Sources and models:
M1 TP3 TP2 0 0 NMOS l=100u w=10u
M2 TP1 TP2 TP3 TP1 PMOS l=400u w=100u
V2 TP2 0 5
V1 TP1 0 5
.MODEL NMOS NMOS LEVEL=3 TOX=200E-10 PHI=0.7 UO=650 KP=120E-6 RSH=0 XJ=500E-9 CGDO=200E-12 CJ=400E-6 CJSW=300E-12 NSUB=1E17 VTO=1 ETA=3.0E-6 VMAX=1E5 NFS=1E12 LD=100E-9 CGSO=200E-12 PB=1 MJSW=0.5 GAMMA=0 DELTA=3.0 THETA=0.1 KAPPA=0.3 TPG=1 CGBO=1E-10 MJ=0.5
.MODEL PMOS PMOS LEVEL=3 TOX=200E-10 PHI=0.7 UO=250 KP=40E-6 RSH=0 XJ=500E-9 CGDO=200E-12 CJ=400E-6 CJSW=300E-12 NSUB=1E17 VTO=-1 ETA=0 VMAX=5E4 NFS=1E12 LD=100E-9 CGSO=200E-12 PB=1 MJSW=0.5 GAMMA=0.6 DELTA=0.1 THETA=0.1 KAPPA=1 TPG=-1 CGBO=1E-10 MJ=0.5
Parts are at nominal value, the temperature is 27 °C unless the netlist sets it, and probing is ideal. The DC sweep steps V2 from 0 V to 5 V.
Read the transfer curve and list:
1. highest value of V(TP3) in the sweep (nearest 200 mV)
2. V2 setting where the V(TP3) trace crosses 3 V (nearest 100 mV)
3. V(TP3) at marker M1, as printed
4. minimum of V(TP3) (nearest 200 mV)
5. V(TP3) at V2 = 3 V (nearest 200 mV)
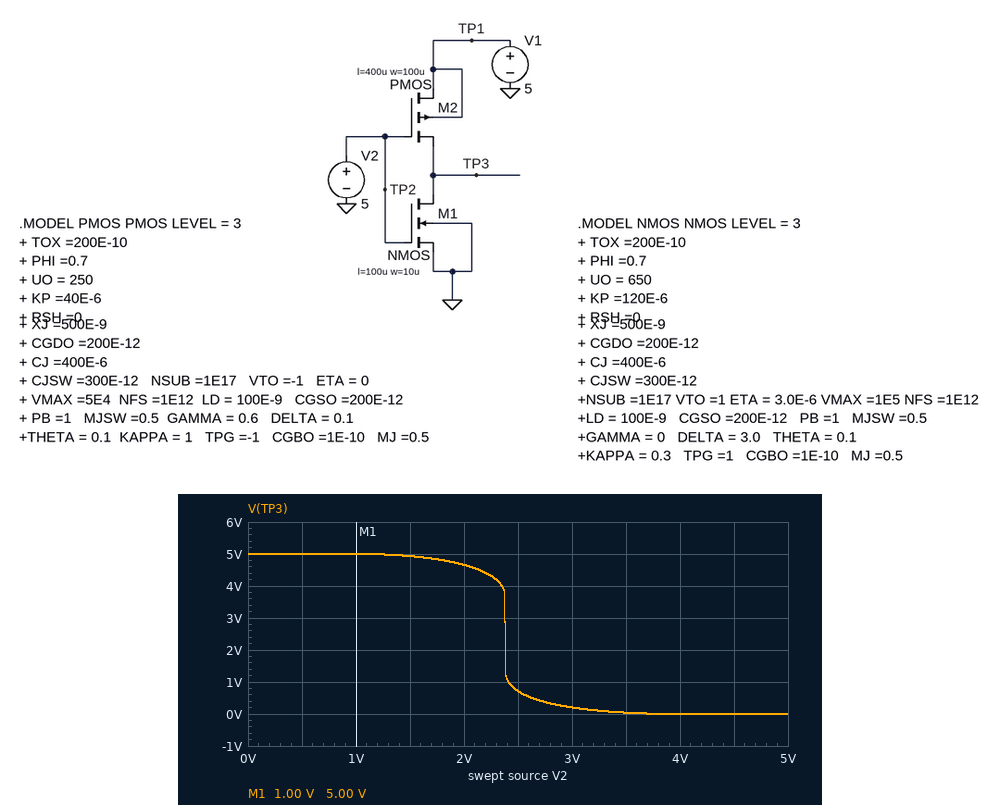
5.0 V
2.4 V
5.00 V
0 V
200 mV
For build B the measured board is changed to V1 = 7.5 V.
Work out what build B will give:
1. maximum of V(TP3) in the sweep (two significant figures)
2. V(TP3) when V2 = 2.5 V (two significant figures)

7.5 V
7.1 V
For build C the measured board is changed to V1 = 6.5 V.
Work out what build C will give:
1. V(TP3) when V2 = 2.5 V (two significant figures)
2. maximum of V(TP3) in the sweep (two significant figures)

6.0 V
6.5 V
